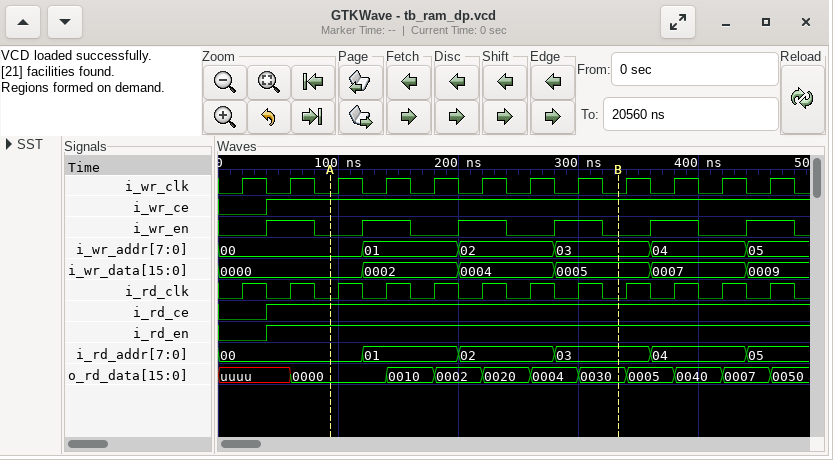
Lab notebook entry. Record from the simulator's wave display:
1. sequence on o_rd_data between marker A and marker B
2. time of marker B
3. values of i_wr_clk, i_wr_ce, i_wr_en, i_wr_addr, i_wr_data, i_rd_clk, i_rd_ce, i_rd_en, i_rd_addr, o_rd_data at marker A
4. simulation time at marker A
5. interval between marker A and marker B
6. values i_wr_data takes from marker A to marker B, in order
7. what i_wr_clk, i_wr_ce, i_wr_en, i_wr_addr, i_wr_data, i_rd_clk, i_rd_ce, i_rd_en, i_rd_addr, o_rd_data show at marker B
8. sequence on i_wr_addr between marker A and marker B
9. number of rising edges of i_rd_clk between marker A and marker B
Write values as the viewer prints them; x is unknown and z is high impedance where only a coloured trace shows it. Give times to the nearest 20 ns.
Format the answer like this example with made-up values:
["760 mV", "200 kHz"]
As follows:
["0000, 0010, 0002, 0020, 0004, 0030", "340 ns", "i_wr_clk=0, i_wr_ce=1, i_wr_en=0, i_wr_addr=00, i_wr_data=0000, i_rd_clk=0, i_rd_ce=1, i_rd_en=1, i_rd_addr=00, o_rd_data=0000", "100 ns", "240 ns", "0000, 0002, 0004, 0005", "i_wr_clk=0, i_wr_ce=1, i_wr_en=0, i_wr_addr=03, i_wr_data=0005, i_rd_clk=0, i_rd_ce=1, i_rd_en=1, i_rd_addr=03, o_rd_data=0030", "00, 01, 02, 03", "6"]
